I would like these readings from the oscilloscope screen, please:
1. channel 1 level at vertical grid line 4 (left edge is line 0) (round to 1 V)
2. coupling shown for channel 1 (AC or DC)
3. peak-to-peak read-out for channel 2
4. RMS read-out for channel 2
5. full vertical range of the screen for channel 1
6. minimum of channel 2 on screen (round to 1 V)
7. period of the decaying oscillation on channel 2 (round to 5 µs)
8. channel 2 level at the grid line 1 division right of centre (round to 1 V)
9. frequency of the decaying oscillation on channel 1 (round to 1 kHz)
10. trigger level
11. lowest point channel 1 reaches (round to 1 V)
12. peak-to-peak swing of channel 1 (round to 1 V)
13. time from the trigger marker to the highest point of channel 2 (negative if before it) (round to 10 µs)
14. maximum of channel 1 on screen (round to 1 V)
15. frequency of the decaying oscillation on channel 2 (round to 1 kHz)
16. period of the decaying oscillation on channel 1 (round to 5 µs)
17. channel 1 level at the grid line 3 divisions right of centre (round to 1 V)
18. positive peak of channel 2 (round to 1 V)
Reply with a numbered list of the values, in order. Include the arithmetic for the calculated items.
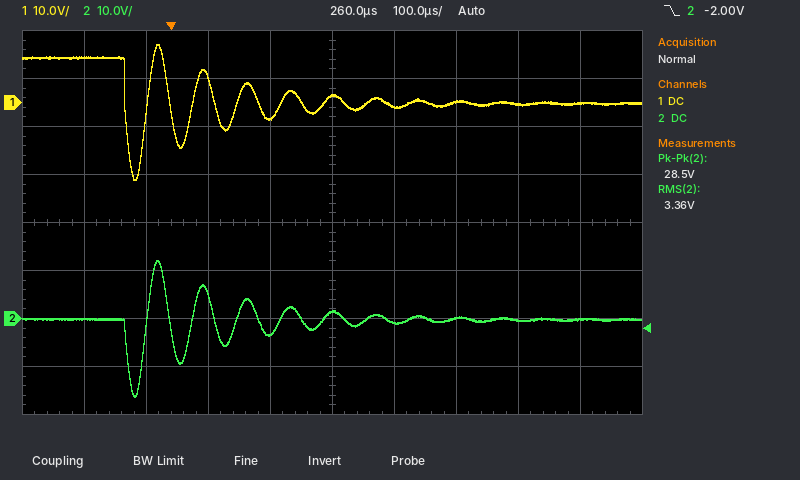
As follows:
1. -3 V
2. DC
3. 28.5 V
4. 3.36 V
5. 80 V
6. -16 V
7. 70 µs
8. -1 V
9. 1 / 70 µs ≈ 14 kHz
10. -2.00 V
11. -16 V
12. 12 V − (-16 V) = 28 V
13. -20 µs
14. 12 V
15. 1 / 70 µs ≈ 14 kHz
16. 70 µs
17. 0 V
18. 12 V
